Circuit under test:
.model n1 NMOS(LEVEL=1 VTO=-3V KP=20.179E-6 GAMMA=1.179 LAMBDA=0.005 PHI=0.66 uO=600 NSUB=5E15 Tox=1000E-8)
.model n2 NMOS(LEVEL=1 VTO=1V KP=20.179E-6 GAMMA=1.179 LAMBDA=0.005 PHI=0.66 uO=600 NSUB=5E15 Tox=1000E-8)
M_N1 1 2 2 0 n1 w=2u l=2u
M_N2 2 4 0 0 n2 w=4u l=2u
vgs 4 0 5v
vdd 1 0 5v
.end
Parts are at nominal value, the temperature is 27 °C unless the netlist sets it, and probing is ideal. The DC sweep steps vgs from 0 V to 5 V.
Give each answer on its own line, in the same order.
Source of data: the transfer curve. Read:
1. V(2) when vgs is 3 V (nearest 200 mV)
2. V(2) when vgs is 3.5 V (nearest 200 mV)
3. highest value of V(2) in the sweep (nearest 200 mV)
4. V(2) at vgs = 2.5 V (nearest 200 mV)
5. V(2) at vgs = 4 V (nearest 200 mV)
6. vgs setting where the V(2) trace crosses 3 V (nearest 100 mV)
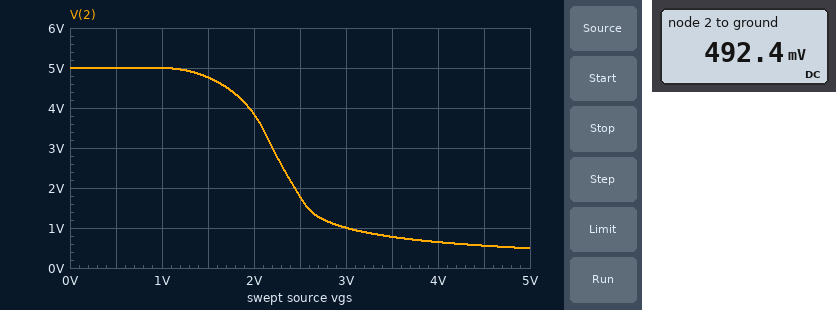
1.0 V
800 mV
5.0 V
1.8 V
600 mV
2.2 V
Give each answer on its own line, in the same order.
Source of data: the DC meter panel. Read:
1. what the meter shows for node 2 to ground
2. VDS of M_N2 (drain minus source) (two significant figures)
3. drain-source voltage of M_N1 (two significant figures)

492.4 mV
490 mV
4.5 V
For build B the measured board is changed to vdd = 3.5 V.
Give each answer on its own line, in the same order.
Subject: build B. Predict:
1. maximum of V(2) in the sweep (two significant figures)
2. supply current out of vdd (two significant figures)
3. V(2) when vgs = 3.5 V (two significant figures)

3.5 V
74 µA
770 mV
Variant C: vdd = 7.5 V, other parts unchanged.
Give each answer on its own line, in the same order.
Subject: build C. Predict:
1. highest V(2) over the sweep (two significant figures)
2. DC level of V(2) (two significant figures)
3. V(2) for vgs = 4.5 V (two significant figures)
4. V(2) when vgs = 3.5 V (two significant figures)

7.5 V
500 mV
560 mV
790 mV
